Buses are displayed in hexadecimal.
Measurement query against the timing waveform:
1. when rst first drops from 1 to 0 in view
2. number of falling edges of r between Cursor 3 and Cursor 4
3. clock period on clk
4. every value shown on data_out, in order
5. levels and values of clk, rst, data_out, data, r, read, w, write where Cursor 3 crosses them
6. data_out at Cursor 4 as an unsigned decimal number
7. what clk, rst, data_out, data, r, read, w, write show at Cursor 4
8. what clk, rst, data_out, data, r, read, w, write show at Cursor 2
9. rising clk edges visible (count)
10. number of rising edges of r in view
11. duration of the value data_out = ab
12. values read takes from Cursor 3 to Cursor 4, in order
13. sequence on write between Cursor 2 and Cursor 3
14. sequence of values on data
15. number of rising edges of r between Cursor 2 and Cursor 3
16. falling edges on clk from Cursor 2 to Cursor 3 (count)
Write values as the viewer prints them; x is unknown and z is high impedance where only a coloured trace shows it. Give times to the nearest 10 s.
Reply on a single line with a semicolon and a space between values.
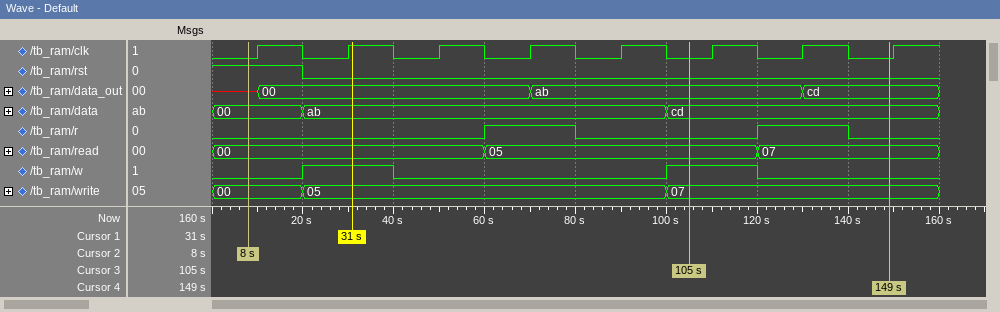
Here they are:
20 s; 1; 20 s; x, 00, ab, cd; clk=0, rst=0, data_out=ab, data=cd, r=0, read=05, w=1, write=07; 205; clk=0, rst=0, data_out=cd, data=cd, r=0, read=07, w=0, write=07; clk=0, rst=1, data_out=x, data=00, r=0, read=00, w=0, write=00; 8; 2; 60 s; 05, 07; 00, 05, 07; 00, ab, cd; 1; 5
